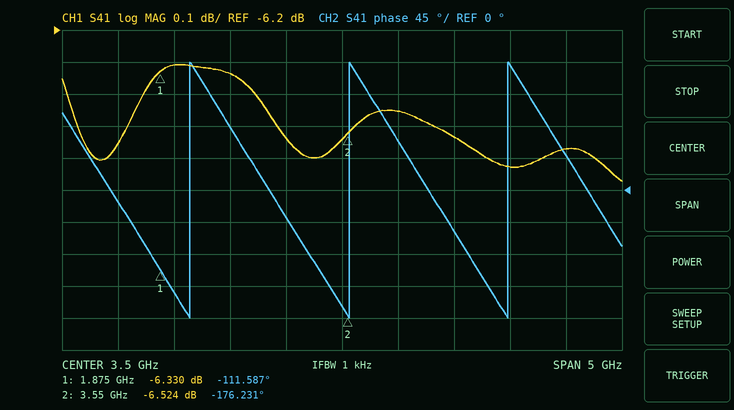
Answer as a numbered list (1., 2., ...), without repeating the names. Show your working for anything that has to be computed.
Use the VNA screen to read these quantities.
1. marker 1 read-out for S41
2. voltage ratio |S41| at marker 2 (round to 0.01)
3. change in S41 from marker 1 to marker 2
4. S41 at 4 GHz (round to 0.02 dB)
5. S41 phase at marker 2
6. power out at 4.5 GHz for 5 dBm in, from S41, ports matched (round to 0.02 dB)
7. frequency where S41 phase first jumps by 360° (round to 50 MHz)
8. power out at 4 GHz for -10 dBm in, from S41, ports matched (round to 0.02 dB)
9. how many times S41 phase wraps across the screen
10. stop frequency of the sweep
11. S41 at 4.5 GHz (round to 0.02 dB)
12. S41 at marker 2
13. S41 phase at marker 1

1. -6.330 dB
2. 10^(-6.524/20) ≈ 0.47
3. -6.524 − (-6.33) = -0.194 dB
4. -6.46 dB
5. -176.231°
6. 5 dBm + (-6.54 dB) = -1.54 dBm
7. 2.15 GHz
8. -10 dBm + (-6.46 dB) = -16.46 dBm
9. 3
10. 6 GHz
11. -6.54 dB
12. -6.524 dB
13. -111.587°
